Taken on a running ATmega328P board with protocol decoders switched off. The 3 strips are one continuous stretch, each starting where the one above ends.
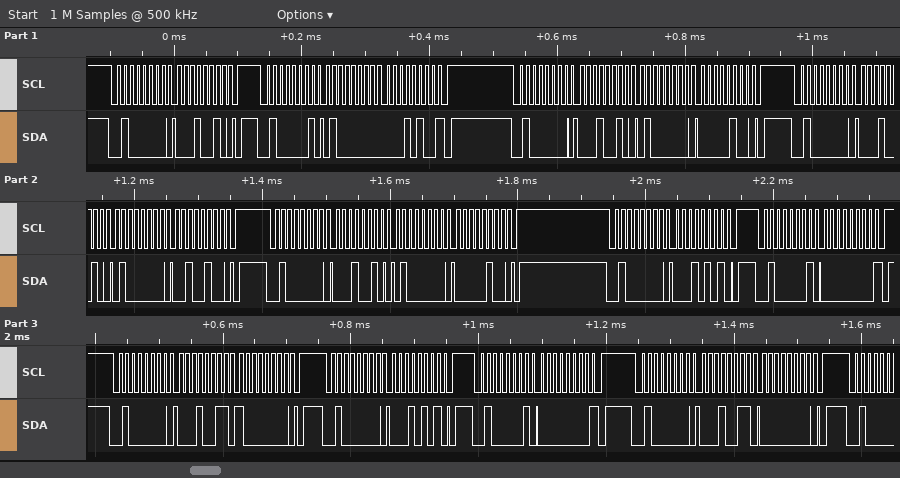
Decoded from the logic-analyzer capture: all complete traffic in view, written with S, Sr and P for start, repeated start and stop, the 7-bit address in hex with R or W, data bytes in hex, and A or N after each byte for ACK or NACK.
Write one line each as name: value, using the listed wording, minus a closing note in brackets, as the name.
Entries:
all complete traffic in view, written with S, Sr and P for start, repeated start and stop, the 7-bit address in hex with R or W, data bytes in hex, and A or N after each byte for ACK or NACK: S 20W A 12 A P S 20R A 40 A 14 N P S 20W A 12 A 40 A 04 A P S 20W A 12 A 40 A 24 A P S 20W A 12 A 40 A 04 A P S 20W A 15 A P S 20R A 00 N P S 20W A 13 A 80 A P S 20W A 15 A P S 20R A 00 N P S 20W A 13 A 00 A P
